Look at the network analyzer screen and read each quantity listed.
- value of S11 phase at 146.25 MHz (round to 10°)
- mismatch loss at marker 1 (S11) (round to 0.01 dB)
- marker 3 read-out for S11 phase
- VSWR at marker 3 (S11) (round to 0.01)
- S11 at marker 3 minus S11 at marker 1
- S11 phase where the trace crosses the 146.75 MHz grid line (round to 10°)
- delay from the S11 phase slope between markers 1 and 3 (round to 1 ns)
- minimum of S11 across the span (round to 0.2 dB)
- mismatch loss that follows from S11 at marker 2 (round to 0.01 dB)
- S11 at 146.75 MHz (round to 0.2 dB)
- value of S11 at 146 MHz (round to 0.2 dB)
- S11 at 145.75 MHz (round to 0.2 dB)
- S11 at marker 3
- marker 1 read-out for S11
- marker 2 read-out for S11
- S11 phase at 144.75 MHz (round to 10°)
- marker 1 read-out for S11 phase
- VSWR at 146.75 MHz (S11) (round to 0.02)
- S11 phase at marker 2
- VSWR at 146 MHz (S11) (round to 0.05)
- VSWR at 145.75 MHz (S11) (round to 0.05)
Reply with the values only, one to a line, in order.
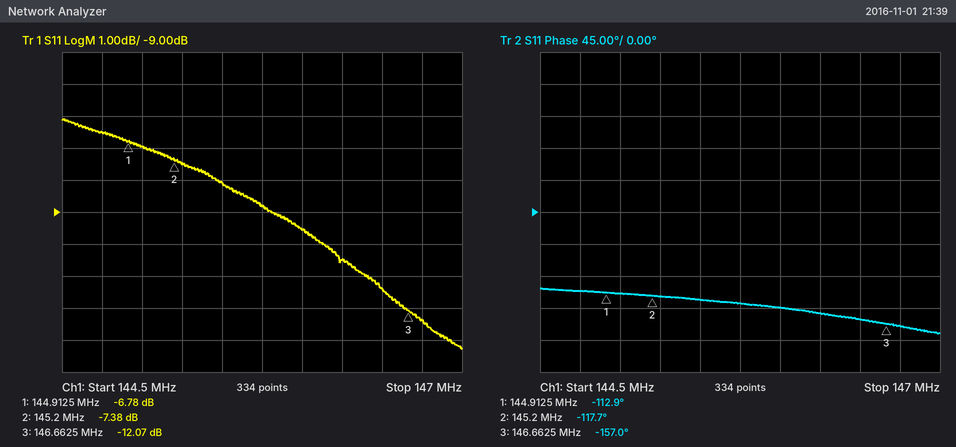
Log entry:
-140°
1.02 dB
-157.0°
1.66
-5.29 dB
-160°
70 ns
-13.2 dB
0.88 dB
-12.4 dB
-9.6 dB
-8.8 dB
-12.07 dB
-6.78 dB
-7.38 dB
-110°
-112.9°
1.64
-117.7°
2.00
2.15
